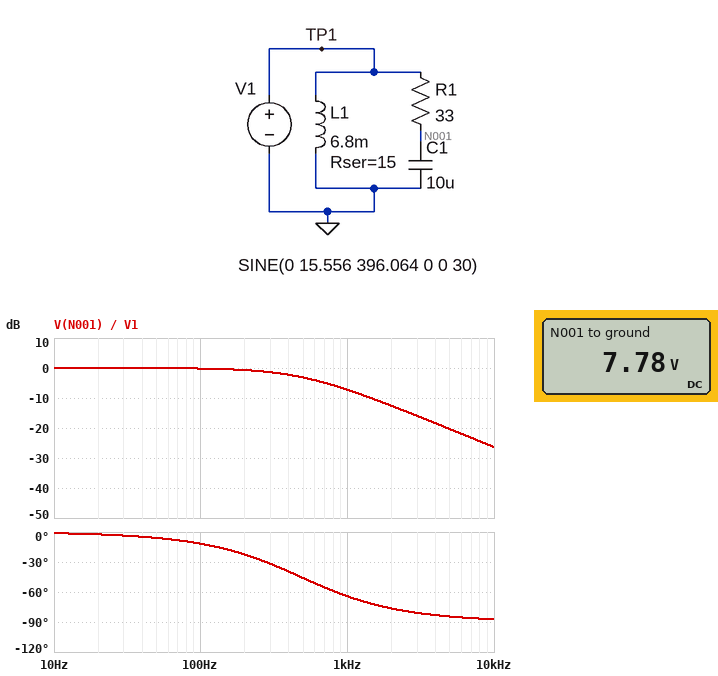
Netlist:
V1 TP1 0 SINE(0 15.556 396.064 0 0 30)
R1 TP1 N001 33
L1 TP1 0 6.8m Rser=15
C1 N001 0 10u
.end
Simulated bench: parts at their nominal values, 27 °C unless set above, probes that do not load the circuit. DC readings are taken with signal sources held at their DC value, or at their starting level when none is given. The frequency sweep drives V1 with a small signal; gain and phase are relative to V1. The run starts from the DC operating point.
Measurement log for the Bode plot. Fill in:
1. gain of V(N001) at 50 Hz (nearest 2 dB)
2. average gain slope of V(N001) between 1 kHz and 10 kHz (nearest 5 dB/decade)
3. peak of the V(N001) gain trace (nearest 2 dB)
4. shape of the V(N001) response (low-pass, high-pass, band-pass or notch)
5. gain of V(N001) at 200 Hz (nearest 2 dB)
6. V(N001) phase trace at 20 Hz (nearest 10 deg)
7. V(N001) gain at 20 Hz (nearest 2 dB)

0 dB
-20 dB/decade
0 dB
low-pass
0 dB
0 deg
0 dB
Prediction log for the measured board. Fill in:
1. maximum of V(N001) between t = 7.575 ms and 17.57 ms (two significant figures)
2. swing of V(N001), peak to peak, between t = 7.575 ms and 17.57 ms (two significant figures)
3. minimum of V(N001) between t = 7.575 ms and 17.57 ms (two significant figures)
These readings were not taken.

12 V
24 V
-12 V
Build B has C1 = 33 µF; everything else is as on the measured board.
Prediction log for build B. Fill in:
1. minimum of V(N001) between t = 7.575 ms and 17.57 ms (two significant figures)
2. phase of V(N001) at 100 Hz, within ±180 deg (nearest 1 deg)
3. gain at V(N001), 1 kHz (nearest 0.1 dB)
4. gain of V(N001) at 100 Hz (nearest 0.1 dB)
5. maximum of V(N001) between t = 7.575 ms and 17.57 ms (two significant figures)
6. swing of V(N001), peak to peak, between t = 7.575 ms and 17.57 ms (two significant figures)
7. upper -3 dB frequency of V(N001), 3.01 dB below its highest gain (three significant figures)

-5.4 V
-34 deg
-16.8 dB
-1.7 dB
5.4 V
11 V
146 Hz
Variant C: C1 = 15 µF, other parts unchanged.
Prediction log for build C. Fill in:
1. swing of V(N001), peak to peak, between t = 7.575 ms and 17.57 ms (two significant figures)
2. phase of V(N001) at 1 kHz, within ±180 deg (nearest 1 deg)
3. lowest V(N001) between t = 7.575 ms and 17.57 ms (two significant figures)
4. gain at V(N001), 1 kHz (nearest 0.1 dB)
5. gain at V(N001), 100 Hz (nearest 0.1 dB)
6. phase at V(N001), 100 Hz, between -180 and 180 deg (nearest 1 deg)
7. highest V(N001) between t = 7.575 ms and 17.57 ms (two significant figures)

20 V
-72 deg
-9.8 V
-10.3 dB
-0.4 dB
-17 deg
9.8 V
